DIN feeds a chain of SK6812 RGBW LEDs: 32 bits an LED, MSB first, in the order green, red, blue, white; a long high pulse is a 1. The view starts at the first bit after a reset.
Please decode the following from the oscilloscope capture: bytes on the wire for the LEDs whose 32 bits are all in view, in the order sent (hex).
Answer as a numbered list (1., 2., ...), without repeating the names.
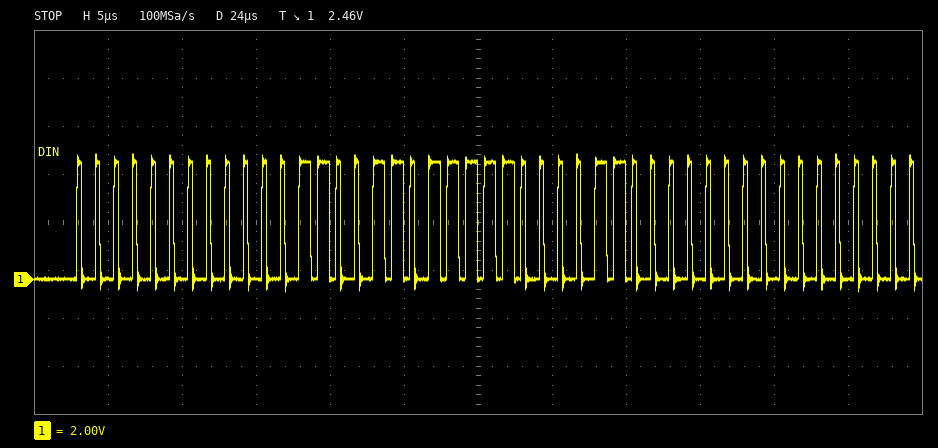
1. 00 0C DF 0C
